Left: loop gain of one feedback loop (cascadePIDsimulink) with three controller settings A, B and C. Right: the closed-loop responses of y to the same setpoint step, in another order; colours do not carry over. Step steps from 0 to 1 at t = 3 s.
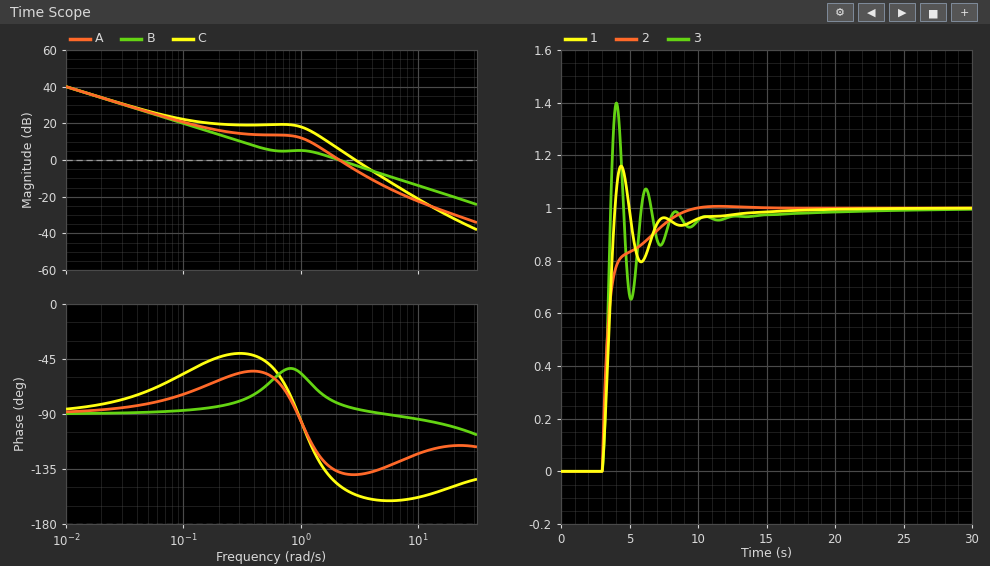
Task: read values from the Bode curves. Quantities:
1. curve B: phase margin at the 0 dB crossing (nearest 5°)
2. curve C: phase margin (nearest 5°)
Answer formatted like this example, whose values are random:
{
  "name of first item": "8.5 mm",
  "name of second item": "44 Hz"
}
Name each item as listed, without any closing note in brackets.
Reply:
{
  "curve B: phase margin at the 0 dB crossing": "100°",
  "curve C: phase margin": "25°"
}
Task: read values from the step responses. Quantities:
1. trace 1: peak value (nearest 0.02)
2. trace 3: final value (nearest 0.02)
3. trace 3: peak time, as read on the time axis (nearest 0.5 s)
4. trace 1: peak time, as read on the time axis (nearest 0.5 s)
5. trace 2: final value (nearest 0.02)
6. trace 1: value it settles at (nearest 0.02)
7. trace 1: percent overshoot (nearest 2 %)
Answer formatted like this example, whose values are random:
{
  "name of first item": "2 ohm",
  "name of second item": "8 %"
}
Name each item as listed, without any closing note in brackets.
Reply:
{
  "trace 1: peak value": "1.16",
  "trace 3: final value": "1.00",
  "trace 3: peak time, as read on the time axis": "4.0 s",
  "trace 1: peak time, as read on the time axis": "4.5 s",
  "trace 2: final value": "1.00",
  "trace 1: value it settles at": "1.00",
  "trace 1: percent overshoot": "16 %"
}
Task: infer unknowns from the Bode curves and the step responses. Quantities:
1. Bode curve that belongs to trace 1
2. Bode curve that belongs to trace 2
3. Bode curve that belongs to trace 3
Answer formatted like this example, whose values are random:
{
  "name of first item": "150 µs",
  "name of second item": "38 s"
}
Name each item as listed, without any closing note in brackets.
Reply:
{
  "Bode curve that belongs to trace 1": "A",
  "Bode curve that belongs to trace 2": "B",
  "Bode curve that belongs to trace 3": "C"
}
